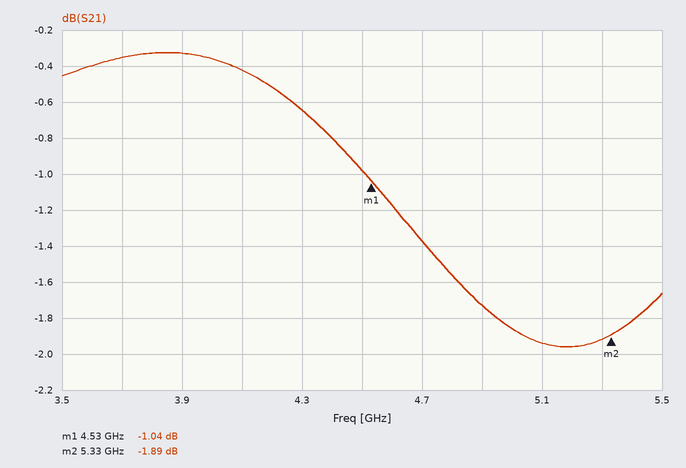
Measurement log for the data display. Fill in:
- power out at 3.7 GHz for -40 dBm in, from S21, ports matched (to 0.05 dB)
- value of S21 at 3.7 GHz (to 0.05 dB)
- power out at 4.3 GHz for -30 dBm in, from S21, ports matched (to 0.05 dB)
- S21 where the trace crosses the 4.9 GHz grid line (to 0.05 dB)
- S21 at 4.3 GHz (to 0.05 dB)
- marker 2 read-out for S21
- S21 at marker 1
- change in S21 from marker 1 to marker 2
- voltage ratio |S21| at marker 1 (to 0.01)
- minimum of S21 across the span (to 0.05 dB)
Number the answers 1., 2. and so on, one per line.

1. -40.35 dBm
2. -0.35 dB
3. -30.65 dBm
4. -1.75 dB
5. -0.65 dB
6. -1.89 dB
7. -1.04 dB
8. -0.85 dB
9. 0.89
10. -1.95 dB
